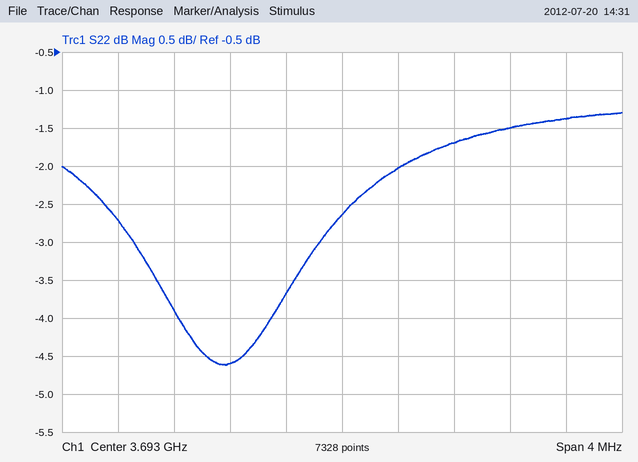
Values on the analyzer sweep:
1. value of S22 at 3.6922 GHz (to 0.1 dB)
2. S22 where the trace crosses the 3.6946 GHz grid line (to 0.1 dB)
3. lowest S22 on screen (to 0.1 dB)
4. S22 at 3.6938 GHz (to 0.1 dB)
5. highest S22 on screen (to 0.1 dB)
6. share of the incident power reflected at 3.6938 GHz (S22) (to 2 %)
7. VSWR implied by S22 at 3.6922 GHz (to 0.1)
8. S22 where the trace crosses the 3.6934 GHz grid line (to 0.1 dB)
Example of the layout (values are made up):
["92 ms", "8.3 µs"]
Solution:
["-4.6 dB", "-1.4 dB", "-4.6 dB", "-1.7 dB", "-1.3 dB", "68 %", "3.9", "-2.0 dB"]
